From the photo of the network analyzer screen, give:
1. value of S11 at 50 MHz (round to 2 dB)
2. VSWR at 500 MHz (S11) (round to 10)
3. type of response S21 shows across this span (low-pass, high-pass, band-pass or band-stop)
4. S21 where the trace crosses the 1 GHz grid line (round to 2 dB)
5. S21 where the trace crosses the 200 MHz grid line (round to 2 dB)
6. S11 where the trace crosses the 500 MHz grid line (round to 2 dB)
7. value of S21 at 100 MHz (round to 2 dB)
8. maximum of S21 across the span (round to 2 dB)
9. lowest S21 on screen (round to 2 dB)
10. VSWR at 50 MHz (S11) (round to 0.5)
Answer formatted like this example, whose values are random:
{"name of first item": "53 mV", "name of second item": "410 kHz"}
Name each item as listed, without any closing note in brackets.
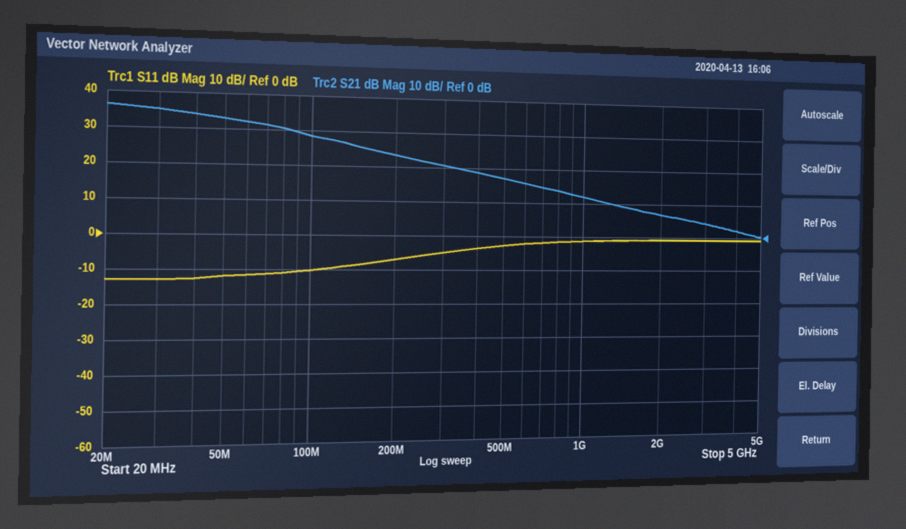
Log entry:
{"value of S11 at 50 MHz": "-12 dB", "VSWR at 500 MHz (S11)": "10", "type of response S21 shows across this span": "low-pass", "S21 where the trace crosses the 1 GHz grid line": "12 dB", "S21 where the trace crosses the 200 MHz grid line": "24 dB", "S11 where the trace crosses the 500 MHz grid line": "-2 dB", "value of S21 at 100 MHz": "28 dB", "maximum of S21 across the span": "36 dB", "lowest S21 on screen": "0 dB", "VSWR at 50 MHz (S11)": "1.5"}
